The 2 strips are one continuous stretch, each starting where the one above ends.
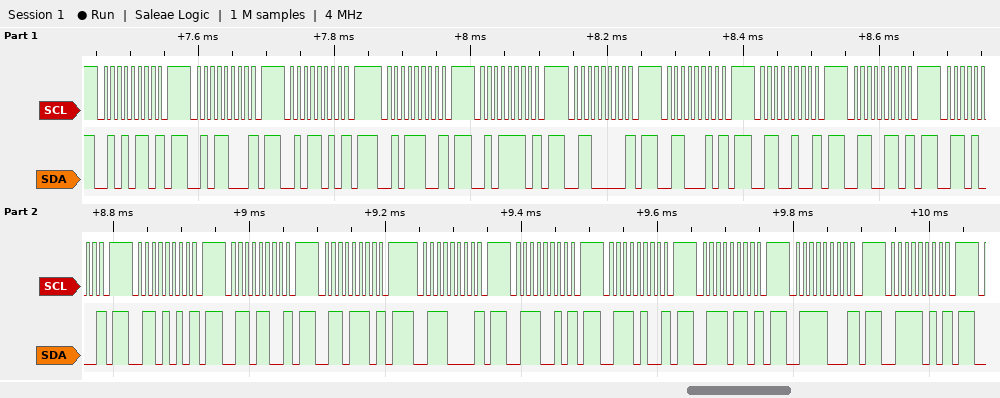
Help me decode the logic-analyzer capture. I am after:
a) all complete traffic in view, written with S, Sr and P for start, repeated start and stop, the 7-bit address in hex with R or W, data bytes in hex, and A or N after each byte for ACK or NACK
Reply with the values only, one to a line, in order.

S 2BW N P S 2CW N P S 2DW N P S 2EW N P S 2FW N P S 30W N P S 31W N P S 32W N P S 33W N P S 34W N P S 35W N P S 36W N P S 37W N P S 38W N P S 39W N P S 3AW N P S 3BW N P S 3CW N P S 3DW N P
